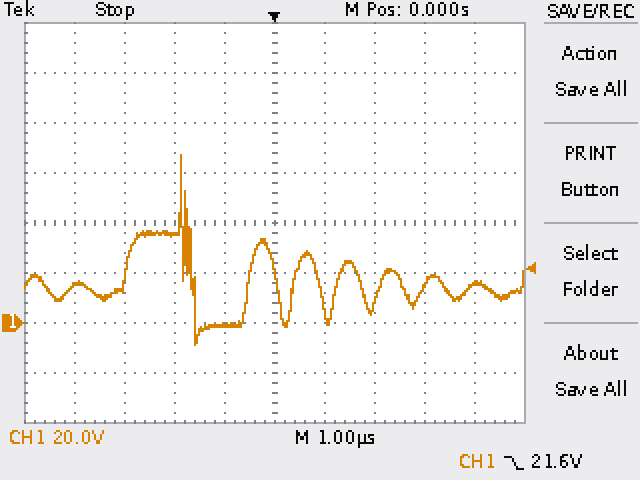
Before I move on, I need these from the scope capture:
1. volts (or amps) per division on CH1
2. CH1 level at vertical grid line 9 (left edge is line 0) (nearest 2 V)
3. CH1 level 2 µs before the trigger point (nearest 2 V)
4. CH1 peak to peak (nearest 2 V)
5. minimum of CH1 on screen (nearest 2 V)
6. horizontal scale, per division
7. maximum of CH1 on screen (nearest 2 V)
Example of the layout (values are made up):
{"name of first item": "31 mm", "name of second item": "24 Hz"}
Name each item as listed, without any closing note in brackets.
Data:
{"volts (or amps) per division on CH1": "20 V", "CH1 level at vertical grid line 9 (left edge is line 0)": "16 V", "CH1 level 2 µs before the trigger point": "36 V", "CH1 peak to peak": "76 V", "minimum of CH1 on screen": "-8 V", "horizontal scale, per division": "1 µs", "maximum of CH1 on screen": "68 V"}
